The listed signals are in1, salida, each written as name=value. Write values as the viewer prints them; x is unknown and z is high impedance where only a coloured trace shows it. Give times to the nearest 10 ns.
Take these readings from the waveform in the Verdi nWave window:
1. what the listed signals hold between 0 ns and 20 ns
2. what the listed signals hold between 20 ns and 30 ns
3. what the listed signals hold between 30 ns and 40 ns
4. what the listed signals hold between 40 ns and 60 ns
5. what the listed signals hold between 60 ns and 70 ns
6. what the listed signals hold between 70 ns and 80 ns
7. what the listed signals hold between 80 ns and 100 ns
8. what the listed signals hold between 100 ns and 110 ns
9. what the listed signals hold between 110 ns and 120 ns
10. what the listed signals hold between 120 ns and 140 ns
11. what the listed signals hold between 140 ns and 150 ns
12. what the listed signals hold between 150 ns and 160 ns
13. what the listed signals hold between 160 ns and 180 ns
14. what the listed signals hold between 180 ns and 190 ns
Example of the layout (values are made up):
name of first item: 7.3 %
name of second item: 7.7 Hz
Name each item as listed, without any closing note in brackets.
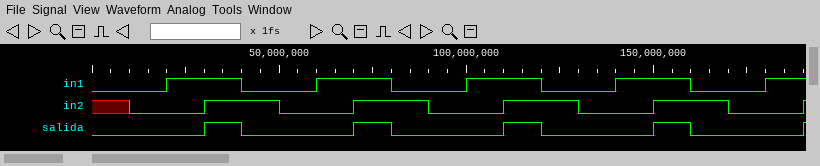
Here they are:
what the listed signals hold between 0 ns and 20 ns: in1=0, salida=0
what the listed signals hold between 20 ns and 30 ns: in1=1, salida=0
what the listed signals hold between 30 ns and 40 ns: in1=1, salida=1
what the listed signals hold between 40 ns and 60 ns: in1=0, salida=0
what the listed signals hold between 60 ns and 70 ns: in1=1, salida=0
what the listed signals hold between 70 ns and 80 ns: in1=1, salida=1
what the listed signals hold between 80 ns and 100 ns: in1=0, salida=0
what the listed signals hold between 100 ns and 110 ns: in1=1, salida=0
what the listed signals hold between 110 ns and 120 ns: in1=1, salida=1
what the listed signals hold between 120 ns and 140 ns: in1=0, salida=0
what the listed signals hold between 140 ns and 150 ns: in1=1, salida=0
what the listed signals hold between 150 ns and 160 ns: in1=1, salida=1
what the listed signals hold between 160 ns and 180 ns: in1=0, salida=0
what the listed signals hold between 180 ns and 190 ns: in1=1, salida=0
